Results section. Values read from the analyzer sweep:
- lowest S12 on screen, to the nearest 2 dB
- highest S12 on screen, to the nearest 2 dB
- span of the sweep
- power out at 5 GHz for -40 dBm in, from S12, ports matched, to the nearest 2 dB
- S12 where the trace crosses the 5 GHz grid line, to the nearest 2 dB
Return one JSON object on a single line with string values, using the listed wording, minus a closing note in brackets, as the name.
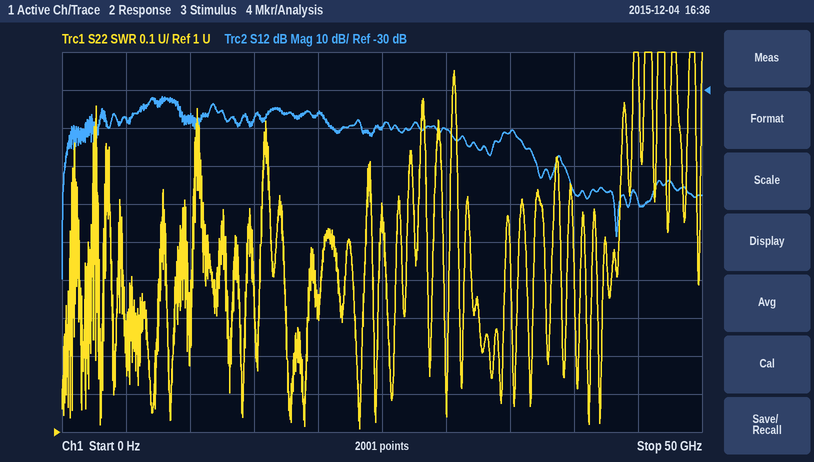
{"lowest S12 on screen, to the nearest 2 dB": "-80 dB", "highest S12 on screen, to the nearest 2 dB": "-32 dB", "span of the sweep": "50 GHz", "power out at 5 GHz for -40 dBm in, from S12, ports matched, to the nearest 2 dB": "-78 dBm", "S12 where the trace crosses the 5 GHz grid line, to the nearest 2 dB": "-38 dB"}
